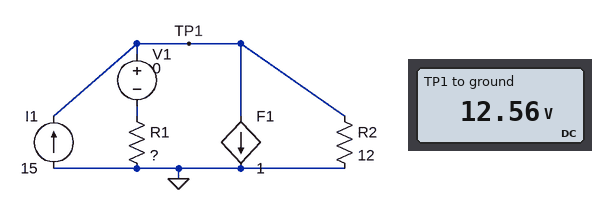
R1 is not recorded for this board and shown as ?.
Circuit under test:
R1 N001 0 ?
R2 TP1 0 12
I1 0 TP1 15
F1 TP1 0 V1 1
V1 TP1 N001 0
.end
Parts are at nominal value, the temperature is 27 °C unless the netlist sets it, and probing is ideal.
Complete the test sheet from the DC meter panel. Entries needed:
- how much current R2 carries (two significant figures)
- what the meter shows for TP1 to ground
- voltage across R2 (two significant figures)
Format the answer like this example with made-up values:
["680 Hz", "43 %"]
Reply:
["1.0 A", "12.56 V", "13 V"]
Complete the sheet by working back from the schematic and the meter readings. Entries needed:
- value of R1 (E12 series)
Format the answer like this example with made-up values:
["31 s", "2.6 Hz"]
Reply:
["1.8 Ω"]
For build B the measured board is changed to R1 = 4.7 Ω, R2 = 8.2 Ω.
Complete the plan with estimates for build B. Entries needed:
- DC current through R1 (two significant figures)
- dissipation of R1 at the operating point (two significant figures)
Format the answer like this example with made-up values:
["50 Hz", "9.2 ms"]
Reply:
["5.8 A", "160 W"]
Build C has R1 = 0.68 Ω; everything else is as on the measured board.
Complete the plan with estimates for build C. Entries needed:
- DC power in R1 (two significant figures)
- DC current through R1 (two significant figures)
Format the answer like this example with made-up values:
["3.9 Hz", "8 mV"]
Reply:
["36 W", "7.3 A"]
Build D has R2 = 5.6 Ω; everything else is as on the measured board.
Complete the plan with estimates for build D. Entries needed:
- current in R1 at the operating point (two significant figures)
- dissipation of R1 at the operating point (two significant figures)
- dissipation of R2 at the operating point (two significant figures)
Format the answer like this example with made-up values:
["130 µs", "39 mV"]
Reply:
["6.5 A", "75 W", "24 W"]
